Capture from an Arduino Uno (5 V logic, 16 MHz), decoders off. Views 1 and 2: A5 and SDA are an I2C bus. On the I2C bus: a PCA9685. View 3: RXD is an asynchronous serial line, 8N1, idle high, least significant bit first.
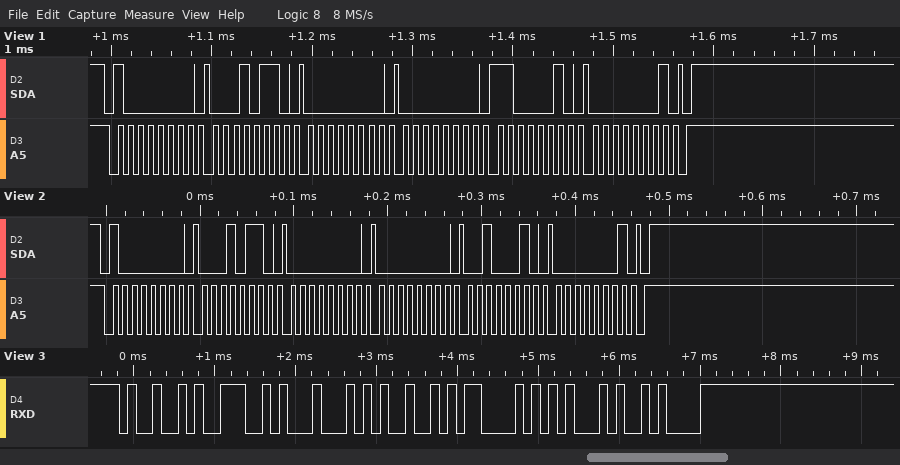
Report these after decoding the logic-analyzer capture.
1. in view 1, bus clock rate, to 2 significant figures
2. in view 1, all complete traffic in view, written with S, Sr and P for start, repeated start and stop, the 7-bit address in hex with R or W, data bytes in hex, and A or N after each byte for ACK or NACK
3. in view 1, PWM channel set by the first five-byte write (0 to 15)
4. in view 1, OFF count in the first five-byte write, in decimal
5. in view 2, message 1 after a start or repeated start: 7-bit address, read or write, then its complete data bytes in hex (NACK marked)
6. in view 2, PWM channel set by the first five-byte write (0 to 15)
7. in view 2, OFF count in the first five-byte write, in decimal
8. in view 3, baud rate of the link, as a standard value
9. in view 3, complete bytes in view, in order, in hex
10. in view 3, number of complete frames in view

100 kHz
S 40W A 16 A 00 A 00 A C2 A 01 A P
4
450
0x40 write: 16 00 00 22 01
4
290
9600 baud
49 4E 44 49 43 45 0A
7
